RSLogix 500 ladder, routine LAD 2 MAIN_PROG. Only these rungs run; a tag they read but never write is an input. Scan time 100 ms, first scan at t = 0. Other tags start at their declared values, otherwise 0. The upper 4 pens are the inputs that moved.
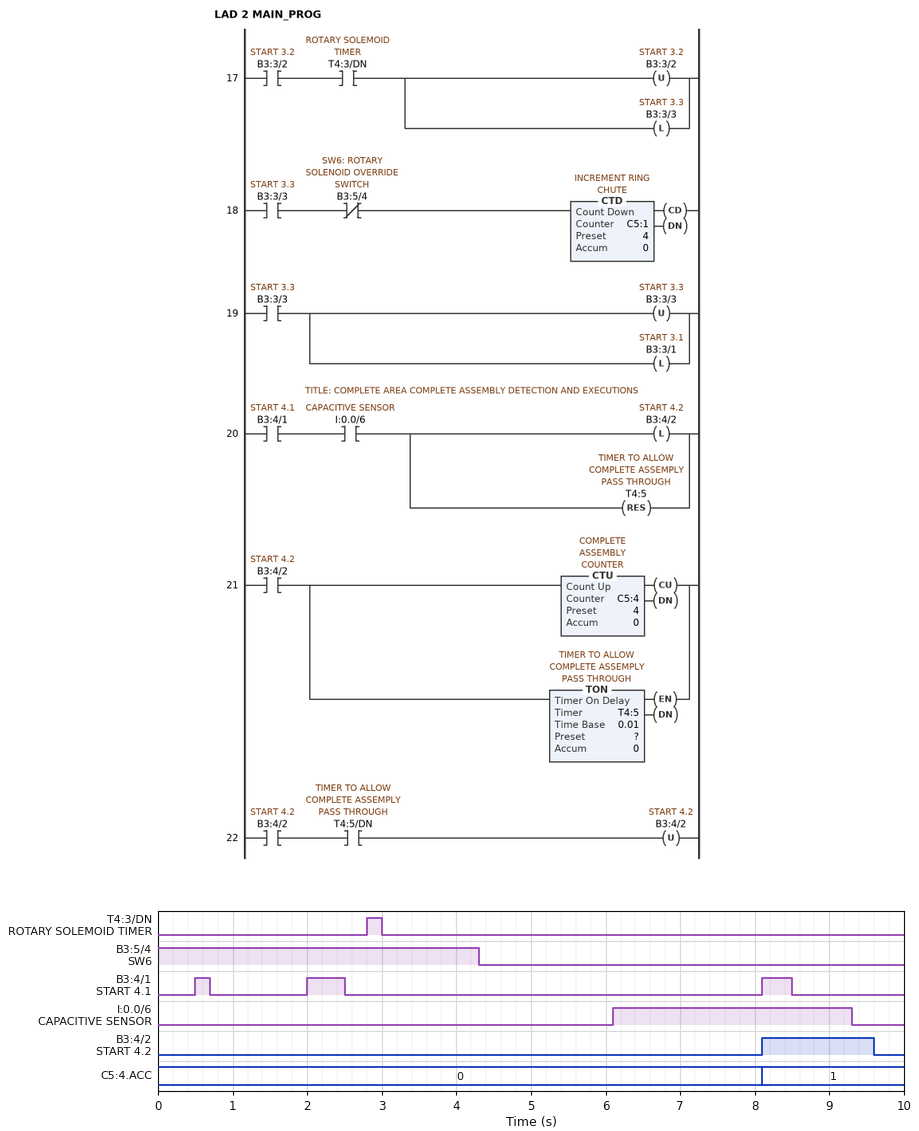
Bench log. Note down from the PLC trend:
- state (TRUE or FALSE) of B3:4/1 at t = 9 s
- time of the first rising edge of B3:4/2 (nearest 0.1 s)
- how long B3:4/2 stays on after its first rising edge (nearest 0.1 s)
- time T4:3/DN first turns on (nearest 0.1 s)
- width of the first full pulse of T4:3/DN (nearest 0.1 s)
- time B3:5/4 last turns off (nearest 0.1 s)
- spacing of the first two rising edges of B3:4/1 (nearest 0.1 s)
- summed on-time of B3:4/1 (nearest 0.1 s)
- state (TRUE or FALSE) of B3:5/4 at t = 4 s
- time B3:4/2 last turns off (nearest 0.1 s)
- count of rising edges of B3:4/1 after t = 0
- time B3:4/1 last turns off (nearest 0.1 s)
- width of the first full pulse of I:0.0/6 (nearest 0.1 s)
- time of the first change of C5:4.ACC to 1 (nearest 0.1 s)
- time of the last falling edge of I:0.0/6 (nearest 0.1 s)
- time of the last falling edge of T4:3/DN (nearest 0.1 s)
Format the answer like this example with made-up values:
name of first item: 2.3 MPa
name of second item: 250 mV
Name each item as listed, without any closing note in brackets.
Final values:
state (TRUE or FALSE) of B3:4/1 at t = 9 s: FALSE
time of the first rising edge of B3:4/2: 8.1 s
how long B3:4/2 stays on after its first rising edge: 1.5 s
time T4:3/DN first turns on: 2.8 s
width of the first full pulse of T4:3/DN: 0.2 s
time B3:5/4 last turns off: 4.3 s
spacing of the first two rising edges of B3:4/1: 1.5 s
summed on-time of B3:4/1: 1.1 s
state (TRUE or FALSE) of B3:5/4 at t = 4 s: TRUE
time B3:4/2 last turns off: 9.6 s
count of rising edges of B3:4/1 after t = 0: 3
time B3:4/1 last turns off: 8.5 s
width of the first full pulse of I:0.0/6: 3.2 s
time of the first change of C5:4.ACC to 1: 8.1 s
time of the last falling edge of I:0.0/6: 9.3 s
time of the last falling edge of T4:3/DN: 3.0 s
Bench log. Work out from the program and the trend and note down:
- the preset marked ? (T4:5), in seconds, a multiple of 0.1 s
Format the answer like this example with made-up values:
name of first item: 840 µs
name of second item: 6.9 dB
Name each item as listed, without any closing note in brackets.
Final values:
the preset marked ? (T4:5), in seconds, a multiple of 0.1 s: 1.2 s
